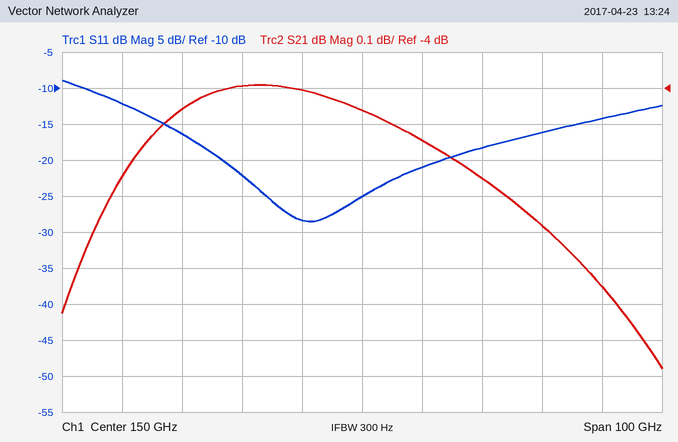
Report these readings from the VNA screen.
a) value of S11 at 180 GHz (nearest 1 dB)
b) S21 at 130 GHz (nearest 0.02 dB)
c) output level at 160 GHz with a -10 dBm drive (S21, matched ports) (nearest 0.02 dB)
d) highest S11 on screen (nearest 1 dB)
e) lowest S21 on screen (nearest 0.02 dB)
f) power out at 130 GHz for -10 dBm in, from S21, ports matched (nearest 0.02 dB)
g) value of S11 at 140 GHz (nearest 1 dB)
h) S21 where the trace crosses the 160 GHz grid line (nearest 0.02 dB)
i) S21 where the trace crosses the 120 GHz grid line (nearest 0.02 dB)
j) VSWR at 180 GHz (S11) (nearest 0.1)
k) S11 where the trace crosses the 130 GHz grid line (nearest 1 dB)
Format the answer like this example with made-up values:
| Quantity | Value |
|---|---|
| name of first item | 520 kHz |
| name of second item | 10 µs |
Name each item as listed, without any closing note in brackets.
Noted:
| Quantity | Value |
|---|---|
| value of S11 at 180 GHz | -16 dB |
| S21 at 130 GHz | -4.00 dB |
| output level at 160 GHz with a -10 dBm drive (S21, matched ports) | -14.14 dBm |
| highest S11 on screen | -9 dB |
| lowest S21 on screen | -4.78 dB |
| power out at 130 GHz for -10 dBm in, from S21, ports matched | -14.00 dBm |
| value of S11 at 140 GHz | -28 dB |
| S21 where the trace crosses the 160 GHz grid line | -4.14 dB |
| S21 where the trace crosses the 120 GHz grid line | -4.06 dB |
| VSWR at 180 GHz (S11) | 1.4 |
| S11 where the trace crosses the 130 GHz grid line | -22 dB |
